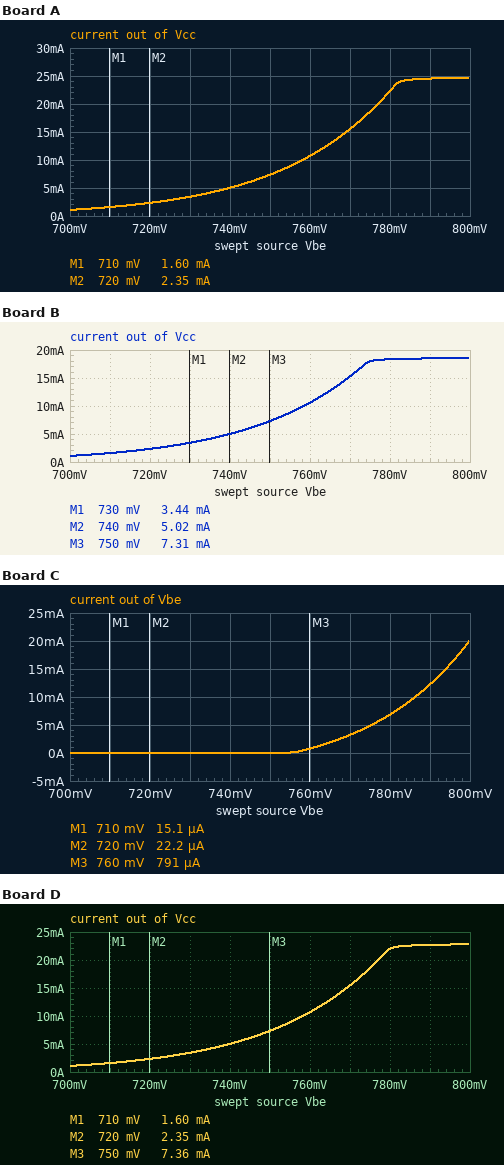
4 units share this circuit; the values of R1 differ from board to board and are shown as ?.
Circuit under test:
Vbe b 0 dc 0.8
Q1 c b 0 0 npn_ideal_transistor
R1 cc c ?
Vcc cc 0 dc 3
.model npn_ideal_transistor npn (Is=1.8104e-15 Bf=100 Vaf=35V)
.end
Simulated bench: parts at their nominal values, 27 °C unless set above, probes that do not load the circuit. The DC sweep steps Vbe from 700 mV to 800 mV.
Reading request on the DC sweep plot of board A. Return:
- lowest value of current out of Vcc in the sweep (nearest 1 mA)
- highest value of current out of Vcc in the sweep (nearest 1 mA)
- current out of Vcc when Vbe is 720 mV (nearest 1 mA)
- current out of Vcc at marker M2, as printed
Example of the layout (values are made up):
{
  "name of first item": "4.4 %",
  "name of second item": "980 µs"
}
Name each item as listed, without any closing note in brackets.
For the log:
{
  "lowest value of current out of Vcc in the sweep": "1 mA",
  "highest value of current out of Vcc in the sweep": "25 mA",
  "current out of Vcc when Vbe is 720 mV": "2 mA",
  "current out of Vcc at marker M2, as printed": "2.35 mA"
}
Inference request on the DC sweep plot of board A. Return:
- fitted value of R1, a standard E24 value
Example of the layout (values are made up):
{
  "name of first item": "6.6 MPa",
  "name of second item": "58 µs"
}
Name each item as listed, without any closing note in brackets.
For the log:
{
  "fitted value of R1, a standard E24 value": "120 Ω"
}
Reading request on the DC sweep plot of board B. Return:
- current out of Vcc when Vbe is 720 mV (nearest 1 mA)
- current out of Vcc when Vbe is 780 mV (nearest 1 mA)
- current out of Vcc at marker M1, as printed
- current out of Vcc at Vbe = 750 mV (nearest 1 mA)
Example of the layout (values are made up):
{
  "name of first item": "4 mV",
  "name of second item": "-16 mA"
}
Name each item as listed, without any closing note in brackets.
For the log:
{
  "current out of Vcc when Vbe is 720 mV": "2 mA",
  "current out of Vcc when Vbe is 780 mV": "18 mA",
  "current out of Vcc at marker M1, as printed": "3.44 mA",
  "current out of Vcc at Vbe = 750 mV": "7 mA"
}
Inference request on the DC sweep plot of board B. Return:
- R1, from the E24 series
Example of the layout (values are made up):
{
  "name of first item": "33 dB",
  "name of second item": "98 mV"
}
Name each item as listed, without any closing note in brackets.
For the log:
{
  "R1, from the E24 series": "160 Ω"
}
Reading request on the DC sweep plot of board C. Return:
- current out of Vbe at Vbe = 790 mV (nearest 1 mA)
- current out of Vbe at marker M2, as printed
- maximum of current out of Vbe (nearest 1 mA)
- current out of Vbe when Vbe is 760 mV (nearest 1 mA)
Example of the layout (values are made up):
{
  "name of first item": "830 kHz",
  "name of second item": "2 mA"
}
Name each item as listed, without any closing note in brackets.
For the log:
{
  "current out of Vbe at Vbe = 790 mV": "12 mA",
  "current out of Vbe at marker M2, as printed": "22.2 µA",
  "maximum of current out of Vbe": "20 mA",
  "current out of Vbe when Vbe is 760 mV": "1 mA"
}
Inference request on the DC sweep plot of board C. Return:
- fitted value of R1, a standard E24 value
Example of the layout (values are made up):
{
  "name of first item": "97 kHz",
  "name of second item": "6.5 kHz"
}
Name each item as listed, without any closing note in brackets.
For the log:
{
  "fitted value of R1, a standard E24 value": "330 Ω"
}
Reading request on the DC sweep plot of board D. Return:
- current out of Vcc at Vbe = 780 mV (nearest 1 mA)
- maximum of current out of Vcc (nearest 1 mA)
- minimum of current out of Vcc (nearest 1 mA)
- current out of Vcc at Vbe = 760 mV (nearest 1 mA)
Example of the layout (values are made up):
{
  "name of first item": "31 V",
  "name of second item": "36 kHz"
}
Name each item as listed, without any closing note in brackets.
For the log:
{
  "current out of Vcc at Vbe = 780 mV": "22 mA",
  "maximum of current out of Vcc": "23 mA",
  "minimum of current out of Vcc": "1 mA",
  "current out of Vcc at Vbe = 760 mV": "11 mA"
}
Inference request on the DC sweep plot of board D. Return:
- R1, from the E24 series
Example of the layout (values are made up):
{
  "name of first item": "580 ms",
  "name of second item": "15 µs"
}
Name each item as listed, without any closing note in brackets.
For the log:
{
  "R1, from the E24 series": "130 Ω"
}
